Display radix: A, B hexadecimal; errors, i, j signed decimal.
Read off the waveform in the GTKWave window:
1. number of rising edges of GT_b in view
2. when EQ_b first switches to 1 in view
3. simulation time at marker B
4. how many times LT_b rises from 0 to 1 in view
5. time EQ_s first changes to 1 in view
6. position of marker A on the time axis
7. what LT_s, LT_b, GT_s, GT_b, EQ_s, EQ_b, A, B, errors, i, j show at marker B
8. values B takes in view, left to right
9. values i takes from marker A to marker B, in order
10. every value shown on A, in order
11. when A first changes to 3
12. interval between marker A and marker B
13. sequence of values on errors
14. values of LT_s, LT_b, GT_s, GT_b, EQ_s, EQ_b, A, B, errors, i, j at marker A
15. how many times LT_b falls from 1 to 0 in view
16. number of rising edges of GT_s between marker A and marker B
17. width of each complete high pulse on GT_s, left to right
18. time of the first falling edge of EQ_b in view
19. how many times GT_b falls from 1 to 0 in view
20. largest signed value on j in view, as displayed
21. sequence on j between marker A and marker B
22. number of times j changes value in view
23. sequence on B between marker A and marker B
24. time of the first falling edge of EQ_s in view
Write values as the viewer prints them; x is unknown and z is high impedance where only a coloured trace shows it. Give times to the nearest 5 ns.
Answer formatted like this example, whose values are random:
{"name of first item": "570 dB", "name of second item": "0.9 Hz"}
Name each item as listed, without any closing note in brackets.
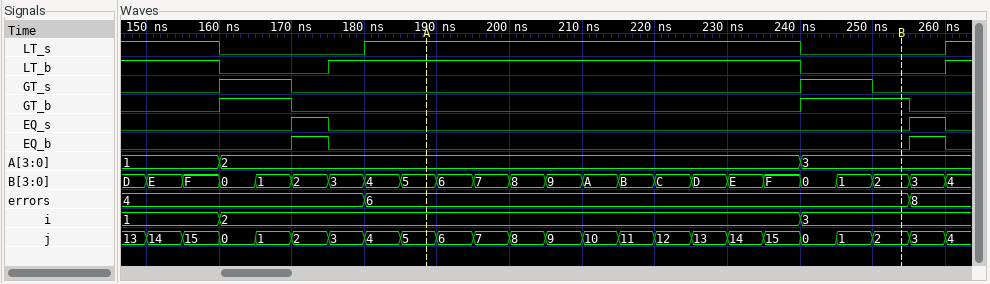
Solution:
{"number of rising edges of GT_b in view": "2", "when EQ_b first switches to 1 in view": "170 ns", "simulation time at marker B": "255 ns", "how many times LT_b rises from 0 to 1 in view": "2", "time EQ_s first changes to 1 in view": "170 ns", "position of marker A on the time axis": "190 ns", "what LT_s, LT_b, GT_s, GT_b, EQ_s, EQ_b, A, B, errors, i, j show at marker B": "LT_s=0, LT_b=0, GT_s=0, GT_b=1, EQ_s=0, EQ_b=0, A=3, B=2, errors=6, i=3, j=2", "values B takes in view, left to right": "D, E, F, 0, 1, 2, 3, 4, 5, 6, 7, 8, 9, A, B, C, D, E, F, 0, 1, 2, 3, 4", "values i takes from marker A to marker B, in order": "2, 3", "every value shown on A, in order": "1, 2, 3", "when A first changes to 3": "240 ns", "interval between marker A and marker B": "65 ns", "sequence of values on errors": "4, 6, 8", "values of LT_s, LT_b, GT_s, GT_b, EQ_s, EQ_b, A, B, errors, i, j at marker A": "LT_s=1, LT_b=1, GT_s=0, GT_b=0, EQ_s=0, EQ_b=0, A=2, B=5, errors=6, i=2, j=5", "how many times LT_b falls from 1 to 0 in view": "2", "number of rising edges of GT_s between marker A and marker B": "1", "width of each complete high pulse on GT_s, left to right": "10 ns, 10 ns", "time of the first falling edge of EQ_b in view": "175 ns", "how many times GT_b falls from 1 to 0 in view": "2", "largest signed value on j in view, as displayed": "15", "sequence on j between marker A and marker B": "5, 6, 7, 8, 9, 10, 11, 12, 13, 14, 15, 0, 1, 2", "number of times j changes value in view": "23", "sequence on B between marker A and marker B": "5, 6, 7, 8, 9, A, B, C, D, E, F, 0, 1, 2", "time of the first falling edge of EQ_s in view": "175 ns"}
